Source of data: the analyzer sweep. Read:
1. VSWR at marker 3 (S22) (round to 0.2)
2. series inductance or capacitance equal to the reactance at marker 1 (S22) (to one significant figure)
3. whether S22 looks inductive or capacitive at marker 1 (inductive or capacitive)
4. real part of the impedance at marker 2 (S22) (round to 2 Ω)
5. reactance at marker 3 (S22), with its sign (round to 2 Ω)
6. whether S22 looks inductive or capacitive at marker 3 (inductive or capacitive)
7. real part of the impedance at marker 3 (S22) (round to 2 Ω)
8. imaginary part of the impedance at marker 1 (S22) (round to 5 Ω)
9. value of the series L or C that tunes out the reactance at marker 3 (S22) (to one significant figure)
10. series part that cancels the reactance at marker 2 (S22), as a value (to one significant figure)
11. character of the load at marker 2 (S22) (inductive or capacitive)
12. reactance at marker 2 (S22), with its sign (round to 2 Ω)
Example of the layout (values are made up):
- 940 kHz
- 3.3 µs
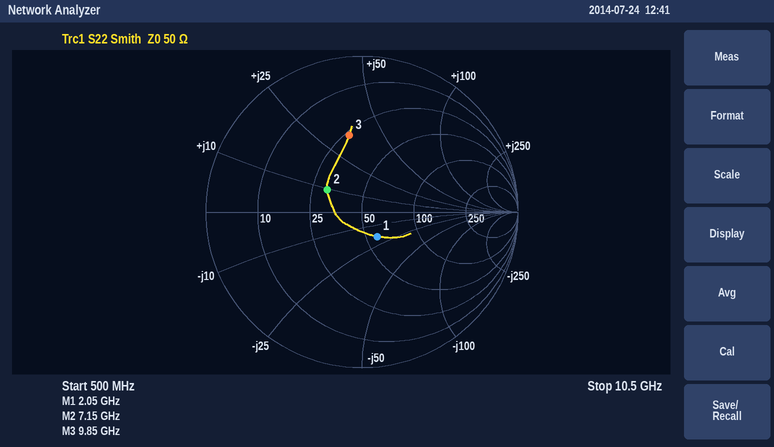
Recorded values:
- 3.0
- 4 pF
- capacitive
- 30 Ω
- +34 Ω
- inductive
- 26 Ω
- -20 Ω
- 500 fF
- 2 pF
- inductive
- +10 Ω
